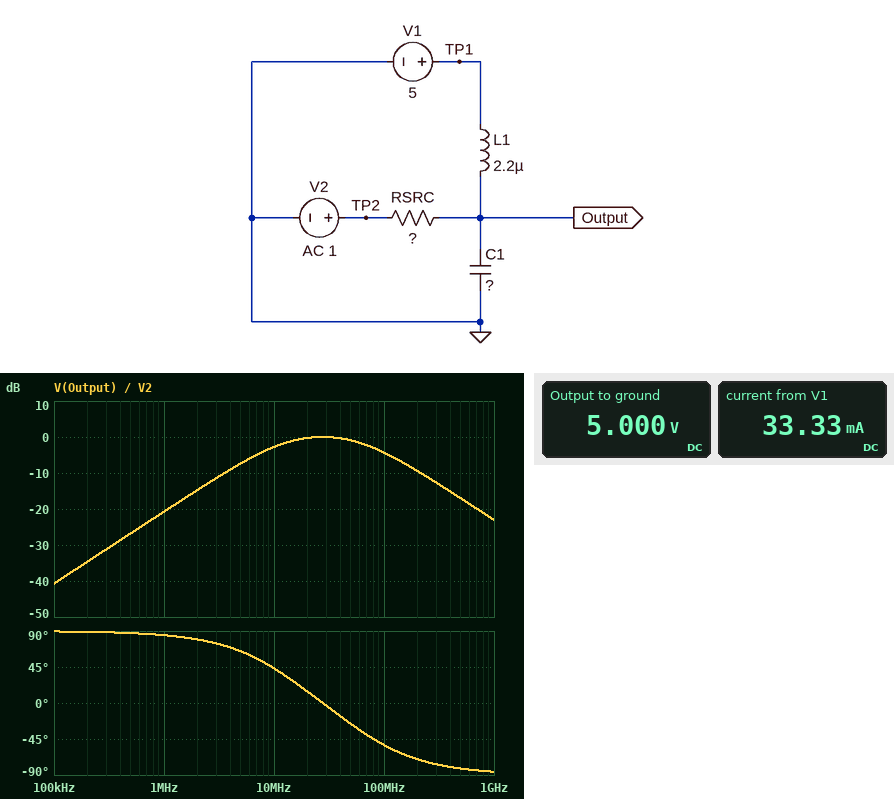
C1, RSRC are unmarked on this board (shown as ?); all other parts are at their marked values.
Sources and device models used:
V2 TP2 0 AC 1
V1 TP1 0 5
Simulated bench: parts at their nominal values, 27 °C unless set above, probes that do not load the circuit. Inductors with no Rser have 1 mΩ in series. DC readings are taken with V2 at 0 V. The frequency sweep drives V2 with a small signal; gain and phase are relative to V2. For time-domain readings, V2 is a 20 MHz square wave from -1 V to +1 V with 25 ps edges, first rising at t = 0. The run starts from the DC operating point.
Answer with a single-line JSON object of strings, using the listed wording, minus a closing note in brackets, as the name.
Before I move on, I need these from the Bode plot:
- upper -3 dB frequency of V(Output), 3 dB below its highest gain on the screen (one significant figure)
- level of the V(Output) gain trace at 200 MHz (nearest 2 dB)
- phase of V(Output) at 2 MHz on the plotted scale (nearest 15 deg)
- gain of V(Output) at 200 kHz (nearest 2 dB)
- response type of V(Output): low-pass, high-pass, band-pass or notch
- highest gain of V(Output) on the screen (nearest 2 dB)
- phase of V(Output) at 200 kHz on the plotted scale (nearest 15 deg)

{"upper -3 dB frequency of V(Output), 3 dB below its highest gain on the screen": "80 MHz", "level of the V(Output) gain trace at 200 MHz": "-10 dB", "phase of V(Output) at 2 MHz on the plotted scale": "75 deg", "gain of V(Output) at 200 kHz": "-34 dB", "response type of V(Output): low-pass, high-pass, band-pass or notch": "band-pass", "highest gain of V(Output) on the screen": "0 dB", "phase of V(Output) at 200 kHz on the plotted scale": "90 deg"}
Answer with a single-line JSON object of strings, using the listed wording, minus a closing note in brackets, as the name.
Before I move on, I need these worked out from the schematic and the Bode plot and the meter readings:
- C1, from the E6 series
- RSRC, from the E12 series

{"C1, from the E6 series": "15 pF", "RSRC, from the E12 series": "150 Ω"}
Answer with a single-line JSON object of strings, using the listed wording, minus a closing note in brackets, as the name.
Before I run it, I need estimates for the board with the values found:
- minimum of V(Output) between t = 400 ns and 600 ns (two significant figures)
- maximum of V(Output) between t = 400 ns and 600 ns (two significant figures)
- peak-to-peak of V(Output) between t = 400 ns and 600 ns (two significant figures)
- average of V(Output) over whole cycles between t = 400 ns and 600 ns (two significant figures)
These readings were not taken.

{"minimum of V(Output) between t = 400 ns and 600 ns": "3.6 V", "maximum of V(Output) between t = 400 ns and 600 ns": "6.4 V", "peak-to-peak of V(Output) between t = 400 ns and 600 ns": "2.7 V", "average of V(Output) over whole cycles between t = 400 ns and 600 ns": "5.0 V"}
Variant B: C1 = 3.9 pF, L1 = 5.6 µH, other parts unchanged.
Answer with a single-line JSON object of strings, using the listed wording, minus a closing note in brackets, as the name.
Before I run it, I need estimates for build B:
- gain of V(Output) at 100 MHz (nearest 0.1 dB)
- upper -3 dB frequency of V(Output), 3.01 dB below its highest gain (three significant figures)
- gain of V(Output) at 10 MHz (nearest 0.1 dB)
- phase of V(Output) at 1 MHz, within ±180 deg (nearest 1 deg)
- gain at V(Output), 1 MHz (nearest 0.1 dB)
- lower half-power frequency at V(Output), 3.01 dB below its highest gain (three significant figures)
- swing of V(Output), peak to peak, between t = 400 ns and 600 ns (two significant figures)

{"gain of V(Output) at 100 MHz": "-0.4 dB", "upper -3 dB frequency of V(Output), 3.01 dB below its highest gain": "276 MHz", "gain of V(Output) at 10 MHz": "-0.6 dB", "phase of V(Output) at 1 MHz, within ±180 deg": "77 deg", "gain at V(Output), 1 MHz": "-12.8 dB", "lower half-power frequency at V(Output), 3.01 dB below its highest gain": "4.20 MHz", "swing of V(Output), peak to peak, between t = 400 ns and 600 ns": "2.5 V"}
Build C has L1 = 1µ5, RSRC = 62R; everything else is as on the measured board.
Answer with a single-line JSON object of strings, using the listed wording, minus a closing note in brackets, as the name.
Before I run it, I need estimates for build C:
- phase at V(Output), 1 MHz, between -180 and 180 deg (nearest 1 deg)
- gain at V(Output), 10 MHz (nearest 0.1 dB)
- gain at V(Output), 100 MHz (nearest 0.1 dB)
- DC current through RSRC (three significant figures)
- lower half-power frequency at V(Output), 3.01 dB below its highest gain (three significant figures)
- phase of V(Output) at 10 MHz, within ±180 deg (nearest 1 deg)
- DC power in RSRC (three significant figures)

{"phase at V(Output), 1 MHz, between -180 and 180 deg": "81 deg", "gain at V(Output), 10 MHz": "-1.3 dB", "gain at V(Output), 100 MHz": "-1.0 dB", "DC current through RSRC": "80.6 mA", "lower half-power frequency at V(Output), 3.01 dB below its highest gain": "6.34 MHz", "phase of V(Output) at 10 MHz, within ±180 deg": "31 deg", "DC power in RSRC": "403 mW"}
